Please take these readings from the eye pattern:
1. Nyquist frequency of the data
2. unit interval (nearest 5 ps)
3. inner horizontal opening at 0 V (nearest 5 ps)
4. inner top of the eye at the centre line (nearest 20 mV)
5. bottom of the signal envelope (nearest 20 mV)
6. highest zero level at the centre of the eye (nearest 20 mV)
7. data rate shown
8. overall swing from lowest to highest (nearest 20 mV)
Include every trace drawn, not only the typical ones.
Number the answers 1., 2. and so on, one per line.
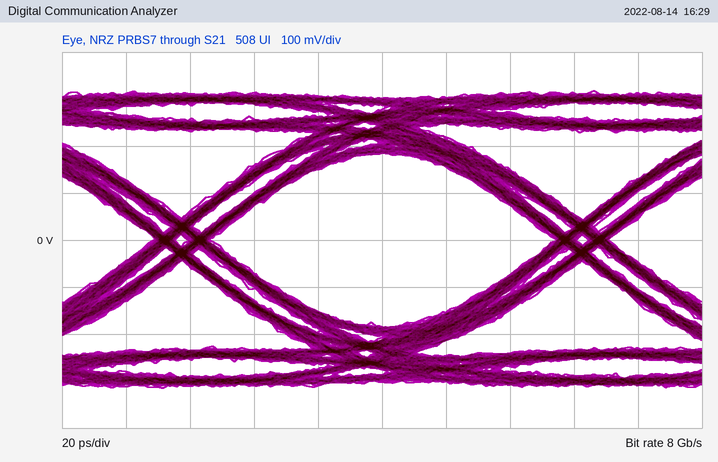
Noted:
1. 4 GHz
2. 125 ps
3. 110 ps
4. 180 mV
5. -320 mV
6. -180 mV
7. 8 Gb/s
8. 640 mV
